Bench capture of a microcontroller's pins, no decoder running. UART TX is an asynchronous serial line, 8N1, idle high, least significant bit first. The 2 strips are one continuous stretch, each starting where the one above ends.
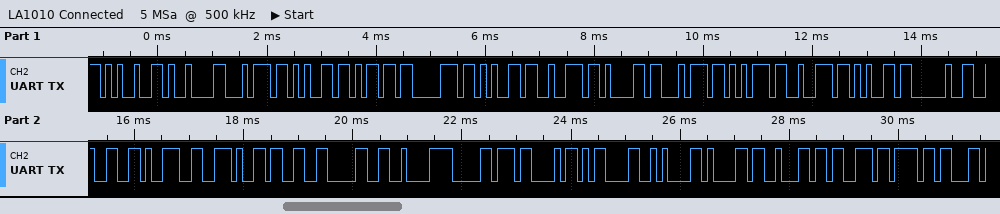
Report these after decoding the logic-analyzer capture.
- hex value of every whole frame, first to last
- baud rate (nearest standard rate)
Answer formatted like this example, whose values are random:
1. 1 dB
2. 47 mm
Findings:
1. 25 09 74 65 6D 70 65 72 61 74 75 72 65 20 32 39 2E 33 30 C2 B0 43 0D 0A 61 62 73 6F
2. 9600 baud
